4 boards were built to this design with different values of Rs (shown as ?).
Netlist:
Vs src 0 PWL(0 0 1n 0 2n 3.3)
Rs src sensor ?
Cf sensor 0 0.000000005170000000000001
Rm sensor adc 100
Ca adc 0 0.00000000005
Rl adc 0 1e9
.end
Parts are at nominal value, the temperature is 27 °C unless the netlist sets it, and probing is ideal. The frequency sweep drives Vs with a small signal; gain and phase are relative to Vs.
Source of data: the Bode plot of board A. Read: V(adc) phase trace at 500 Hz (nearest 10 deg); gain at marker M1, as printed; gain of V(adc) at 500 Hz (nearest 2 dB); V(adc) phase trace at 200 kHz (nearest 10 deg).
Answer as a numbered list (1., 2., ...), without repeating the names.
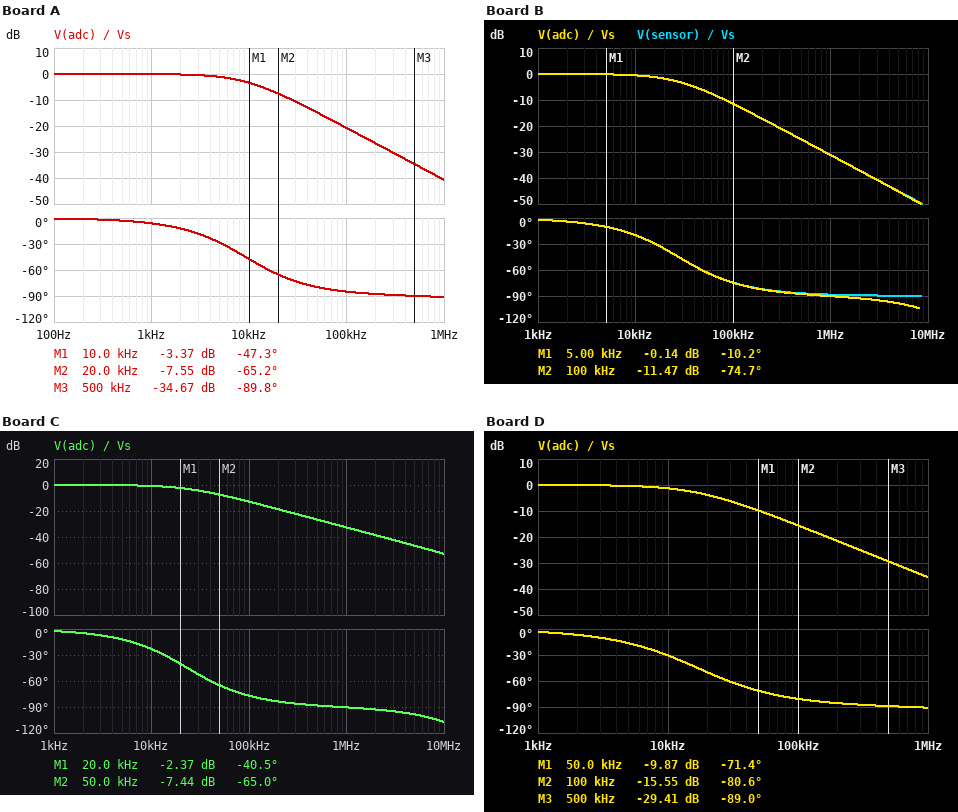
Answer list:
1. 0 deg
2. -3.37 dB
3. 0 dB
4. -90 deg
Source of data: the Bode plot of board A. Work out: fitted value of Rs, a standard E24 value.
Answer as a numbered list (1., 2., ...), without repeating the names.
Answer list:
1. 3.3 kΩ
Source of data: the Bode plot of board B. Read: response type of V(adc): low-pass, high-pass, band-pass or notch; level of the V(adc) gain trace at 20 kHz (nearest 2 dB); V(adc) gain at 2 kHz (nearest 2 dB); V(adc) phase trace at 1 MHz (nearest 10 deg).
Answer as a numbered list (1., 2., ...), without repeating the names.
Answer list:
1. low-pass
2. -2 dB
3. 0 dB
4. -90 deg
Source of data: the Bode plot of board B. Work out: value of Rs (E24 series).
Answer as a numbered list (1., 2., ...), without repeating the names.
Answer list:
1. 1.1 kΩ
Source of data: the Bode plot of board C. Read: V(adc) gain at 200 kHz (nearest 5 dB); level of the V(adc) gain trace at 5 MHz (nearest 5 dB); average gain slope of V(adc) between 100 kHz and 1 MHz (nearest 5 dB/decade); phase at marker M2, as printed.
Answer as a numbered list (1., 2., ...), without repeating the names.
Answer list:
1. -20 dB
2. -45 dB
3. -20 dB/decade
4. -65.0 deg
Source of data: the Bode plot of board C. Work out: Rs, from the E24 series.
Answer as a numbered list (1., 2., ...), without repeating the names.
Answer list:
1. 1.3 kΩ
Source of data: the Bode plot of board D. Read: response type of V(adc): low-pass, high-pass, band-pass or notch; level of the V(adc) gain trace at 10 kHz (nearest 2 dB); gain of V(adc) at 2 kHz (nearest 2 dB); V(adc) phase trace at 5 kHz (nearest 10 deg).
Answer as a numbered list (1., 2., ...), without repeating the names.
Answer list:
1. low-pass
2. -2 dB
3. 0 dB
4. -20 deg
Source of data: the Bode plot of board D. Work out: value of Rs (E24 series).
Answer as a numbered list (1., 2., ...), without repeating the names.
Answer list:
1. 1.8 kΩ
